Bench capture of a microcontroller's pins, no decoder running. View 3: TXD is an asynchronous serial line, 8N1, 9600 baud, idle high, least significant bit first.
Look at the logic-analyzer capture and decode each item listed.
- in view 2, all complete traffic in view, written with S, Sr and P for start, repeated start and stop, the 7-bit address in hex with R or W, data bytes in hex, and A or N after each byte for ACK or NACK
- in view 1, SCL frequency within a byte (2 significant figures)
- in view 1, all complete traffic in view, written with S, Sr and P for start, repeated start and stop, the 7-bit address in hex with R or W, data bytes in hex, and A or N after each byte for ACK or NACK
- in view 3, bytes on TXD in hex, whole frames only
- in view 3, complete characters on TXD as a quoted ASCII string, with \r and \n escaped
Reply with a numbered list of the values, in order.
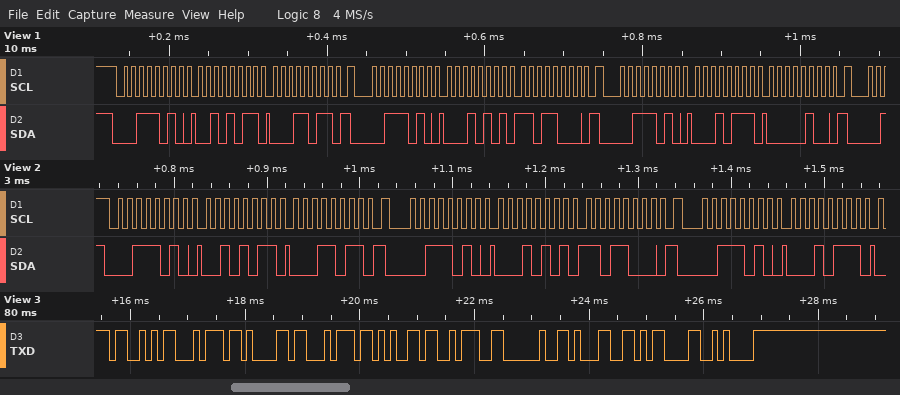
1. S 1DW A 2B A 1B A Sr 1DW A 15 A D8 A Sr 1DW A 17 A
2. 100 kHz
3. S 1DW A 2B A 1B A Sr 1DW A 15 A D8 A Sr 1DW A 17 A 04 A
4. 0x53 0x74 0x61 0x74 0x65 0x3A 0x20 0x31 0x0D 0x0A
5. "State: 1\r\n"
